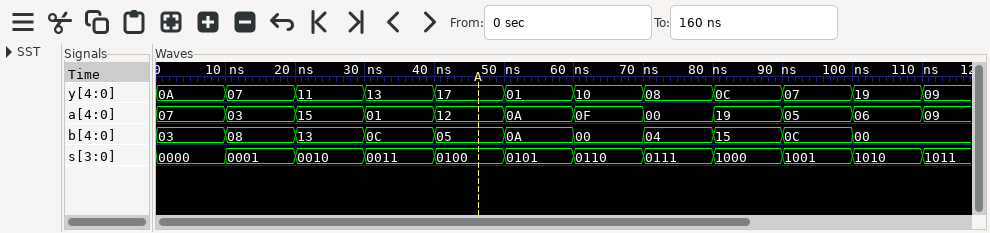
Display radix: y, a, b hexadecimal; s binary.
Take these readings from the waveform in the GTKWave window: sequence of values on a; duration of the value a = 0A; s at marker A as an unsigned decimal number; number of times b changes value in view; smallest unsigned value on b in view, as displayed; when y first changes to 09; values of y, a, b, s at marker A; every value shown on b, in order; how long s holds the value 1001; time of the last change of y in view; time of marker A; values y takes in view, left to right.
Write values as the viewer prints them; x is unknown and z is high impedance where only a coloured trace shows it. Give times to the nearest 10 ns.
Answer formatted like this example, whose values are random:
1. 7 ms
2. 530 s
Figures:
1. 07, 03, 15, 01, 12, 0A, 0F, 00, 19, 05, 06, 09
2. 10 ns
3. 4
4. 10
5. 00
6. 110 ns
7. y=17, a=12, b=05, s=0100
8. 03, 08, 13, 0C, 05, 0A, 00, 04, 15, 0C, 00
9. 10 ns
10. 110 ns
11. 50 ns
12. 0A, 07, 11, 13, 17, 01, 10, 08, 0C, 07, 19, 09
